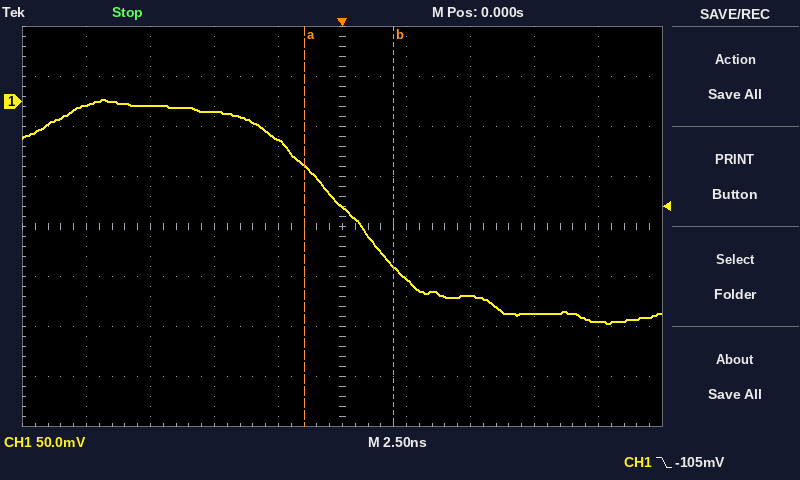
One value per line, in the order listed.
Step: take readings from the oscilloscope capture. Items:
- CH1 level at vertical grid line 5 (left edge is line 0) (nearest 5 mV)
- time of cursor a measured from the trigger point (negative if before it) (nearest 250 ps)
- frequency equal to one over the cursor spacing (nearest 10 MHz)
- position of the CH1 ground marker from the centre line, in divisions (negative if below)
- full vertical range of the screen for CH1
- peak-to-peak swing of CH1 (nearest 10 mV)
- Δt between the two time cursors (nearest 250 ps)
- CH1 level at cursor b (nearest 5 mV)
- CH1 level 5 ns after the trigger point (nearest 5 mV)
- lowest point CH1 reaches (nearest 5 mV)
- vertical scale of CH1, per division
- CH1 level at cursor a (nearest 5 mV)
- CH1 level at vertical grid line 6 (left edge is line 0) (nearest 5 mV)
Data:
-105 mV
-1.50 ns
290 MHz
+2.5 div
400 mV
220 mV
3.50 ns
-165 mV
-195 mV
-220 mV
50 mV
-65 mV
-175 mV
